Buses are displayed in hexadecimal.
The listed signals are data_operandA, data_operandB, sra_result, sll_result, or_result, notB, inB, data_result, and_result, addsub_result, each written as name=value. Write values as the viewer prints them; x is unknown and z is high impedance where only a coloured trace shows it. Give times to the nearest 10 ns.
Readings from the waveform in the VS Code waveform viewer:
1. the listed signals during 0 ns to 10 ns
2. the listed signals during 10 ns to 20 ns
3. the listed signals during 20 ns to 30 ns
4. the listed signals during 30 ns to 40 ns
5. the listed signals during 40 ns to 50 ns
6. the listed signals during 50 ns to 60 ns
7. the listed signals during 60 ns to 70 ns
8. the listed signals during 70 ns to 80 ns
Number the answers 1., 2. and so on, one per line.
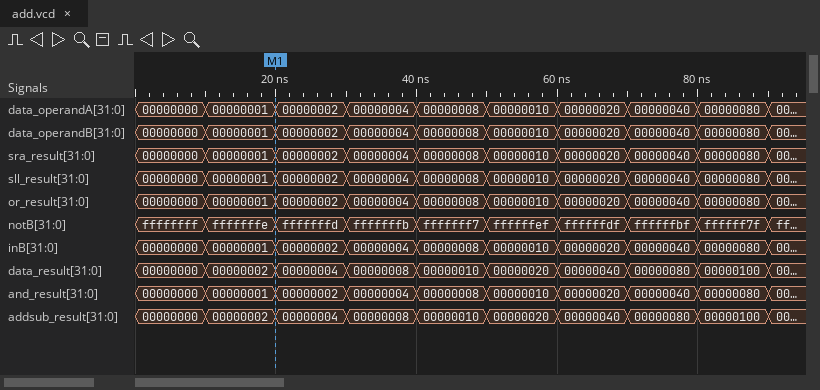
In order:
1. data_operandA=00000000, data_operandB=00000000, sra_result=00000000, sll_result=00000000, or_result=00000000, notB=ffffffff, inB=00000000, data_result=00000000, and_result=00000000, addsub_result=00000000
2. data_operandA=00000001, data_operandB=00000001, sra_result=00000001, sll_result=00000001, or_result=00000001, notB=fffffffe, inB=00000001, data_result=00000002, and_result=00000001, addsub_result=00000002
3. data_operandA=00000002, data_operandB=00000002, sra_result=00000002, sll_result=00000002, or_result=00000002, notB=fffffffd, inB=00000002, data_result=00000004, and_result=00000002, addsub_result=00000004
4. data_operandA=00000004, data_operandB=00000004, sra_result=00000004, sll_result=00000004, or_result=00000004, notB=fffffffb, inB=00000004, data_result=00000008, and_result=00000004, addsub_result=00000008
5. data_operandA=00000008, data_operandB=00000008, sra_result=00000008, sll_result=00000008, or_result=00000008, notB=fffffff7, inB=00000008, data_result=00000010, and_result=00000008, addsub_result=00000010
6. data_operandA=00000010, data_operandB=00000010, sra_result=00000010, sll_result=00000010, or_result=00000010, notB=ffffffef, inB=00000010, data_result=00000020, and_result=00000010, addsub_result=00000020
7. data_operandA=00000020, data_operandB=00000020, sra_result=00000020, sll_result=00000020, or_result=00000020, notB=ffffffdf, inB=00000020, data_result=00000040, and_result=00000020, addsub_result=00000040
8. data_operandA=00000040, data_operandB=00000040, sra_result=00000040, sll_result=00000040, or_result=00000040, notB=ffffffbf, inB=00000040, data_result=00000080, and_result=00000040, addsub_result=00000080
